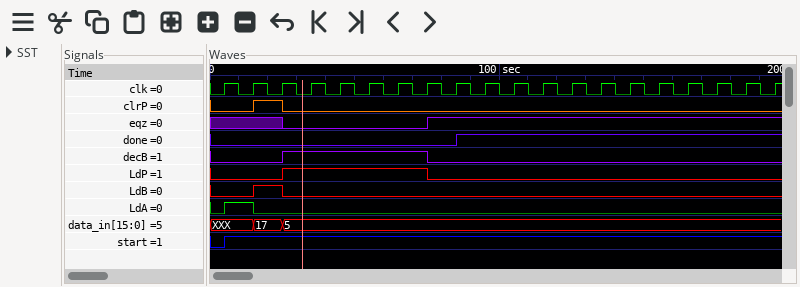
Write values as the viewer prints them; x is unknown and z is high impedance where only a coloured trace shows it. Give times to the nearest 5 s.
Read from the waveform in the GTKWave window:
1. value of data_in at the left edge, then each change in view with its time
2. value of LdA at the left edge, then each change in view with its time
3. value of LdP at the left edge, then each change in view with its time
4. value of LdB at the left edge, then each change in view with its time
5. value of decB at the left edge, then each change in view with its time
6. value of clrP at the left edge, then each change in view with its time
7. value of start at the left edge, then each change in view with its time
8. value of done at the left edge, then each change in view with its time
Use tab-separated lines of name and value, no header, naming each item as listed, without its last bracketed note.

value of data_in at the left edge, then each change in view with its time	XXX, 17 at 15 s, 5 at 25 s
value of LdA at the left edge, then each change in view with its time	0, 1 at 5 s, 0 at 15 s
value of LdP at the left edge, then each change in view with its time	0, 1 at 25 s, 0 at 75 s
value of LdB at the left edge, then each change in view with its time	0, 1 at 15 s, 0 at 25 s
value of decB at the left edge, then each change in view with its time	0, 1 at 25 s, 0 at 75 s
value of clrP at the left edge, then each change in view with its time	0, 1 at 15 s, 0 at 25 s
value of start at the left edge, then each change in view with its time	0, 1 at 5 s
value of done at the left edge, then each change in view with its time	0, 1 at 85 s
